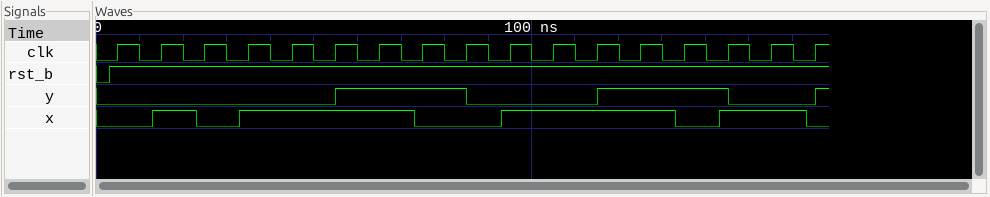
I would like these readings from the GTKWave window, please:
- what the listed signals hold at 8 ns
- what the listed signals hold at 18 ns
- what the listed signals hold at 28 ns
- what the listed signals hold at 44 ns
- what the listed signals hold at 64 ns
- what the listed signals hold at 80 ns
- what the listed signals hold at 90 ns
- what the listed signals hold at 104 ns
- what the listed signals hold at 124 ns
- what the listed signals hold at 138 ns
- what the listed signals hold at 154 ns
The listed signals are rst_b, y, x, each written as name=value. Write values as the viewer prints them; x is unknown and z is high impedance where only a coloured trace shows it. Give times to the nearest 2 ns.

rst_b=1, y=0, x=0
rst_b=1, y=0, x=1
rst_b=1, y=0, x=0
rst_b=1, y=0, x=1
rst_b=1, y=1, x=1
rst_b=1, y=1, x=0
rst_b=1, y=0, x=0
rst_b=1, y=0, x=1
rst_b=1, y=1, x=1
rst_b=1, y=1, x=0
rst_b=1, y=0, x=1
